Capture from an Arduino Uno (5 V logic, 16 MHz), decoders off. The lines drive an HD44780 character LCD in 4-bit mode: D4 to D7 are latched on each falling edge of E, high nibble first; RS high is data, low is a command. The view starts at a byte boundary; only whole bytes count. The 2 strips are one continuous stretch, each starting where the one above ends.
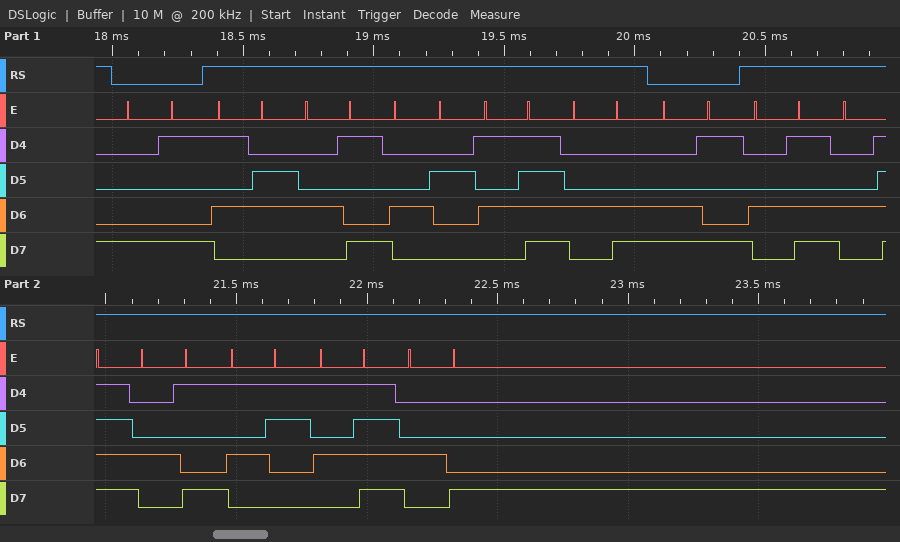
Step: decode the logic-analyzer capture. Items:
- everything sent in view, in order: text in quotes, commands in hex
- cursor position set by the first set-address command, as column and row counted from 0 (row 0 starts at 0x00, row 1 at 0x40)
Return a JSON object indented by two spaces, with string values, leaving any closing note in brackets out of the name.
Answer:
{
  "everything sent in view, in order: text in quotes, commands in hex": "0x89 \"VIB_L\" 0xC9 \"MOIS_H\"",
  "cursor position set by the first set-address command, as column and row counted from 0": "column 9, row 0"
}
